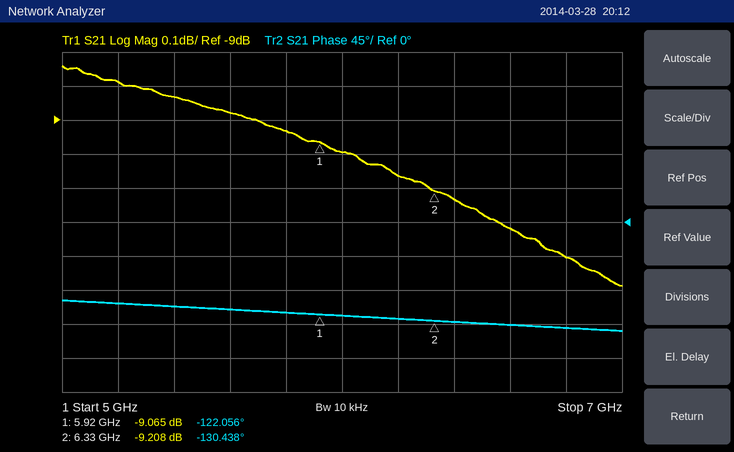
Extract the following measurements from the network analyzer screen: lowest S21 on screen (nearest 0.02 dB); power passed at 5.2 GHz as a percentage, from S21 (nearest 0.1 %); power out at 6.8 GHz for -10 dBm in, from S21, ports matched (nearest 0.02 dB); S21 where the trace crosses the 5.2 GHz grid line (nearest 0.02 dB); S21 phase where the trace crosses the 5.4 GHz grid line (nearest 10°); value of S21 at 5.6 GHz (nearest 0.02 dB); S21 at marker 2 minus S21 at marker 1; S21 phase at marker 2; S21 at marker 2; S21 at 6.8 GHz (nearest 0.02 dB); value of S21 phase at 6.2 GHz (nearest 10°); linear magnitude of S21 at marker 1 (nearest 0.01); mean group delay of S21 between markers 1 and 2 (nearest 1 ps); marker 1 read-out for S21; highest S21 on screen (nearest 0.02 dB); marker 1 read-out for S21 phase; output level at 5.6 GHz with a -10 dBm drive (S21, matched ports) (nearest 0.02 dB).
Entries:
-9.48 dB
12.9 %
-19.40 dBm
-8.88 dB
-110°
-8.98 dB
-0.143 dB
-130.438°
-9.208 dB
-9.40 dB
-130°
0.35
57 ps
-9.065 dB
-8.84 dB
-122.056°
-18.98 dBm
